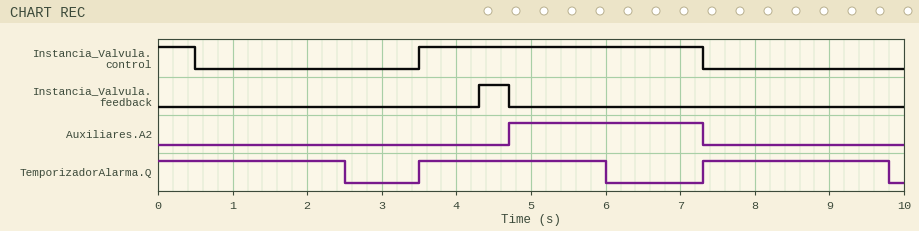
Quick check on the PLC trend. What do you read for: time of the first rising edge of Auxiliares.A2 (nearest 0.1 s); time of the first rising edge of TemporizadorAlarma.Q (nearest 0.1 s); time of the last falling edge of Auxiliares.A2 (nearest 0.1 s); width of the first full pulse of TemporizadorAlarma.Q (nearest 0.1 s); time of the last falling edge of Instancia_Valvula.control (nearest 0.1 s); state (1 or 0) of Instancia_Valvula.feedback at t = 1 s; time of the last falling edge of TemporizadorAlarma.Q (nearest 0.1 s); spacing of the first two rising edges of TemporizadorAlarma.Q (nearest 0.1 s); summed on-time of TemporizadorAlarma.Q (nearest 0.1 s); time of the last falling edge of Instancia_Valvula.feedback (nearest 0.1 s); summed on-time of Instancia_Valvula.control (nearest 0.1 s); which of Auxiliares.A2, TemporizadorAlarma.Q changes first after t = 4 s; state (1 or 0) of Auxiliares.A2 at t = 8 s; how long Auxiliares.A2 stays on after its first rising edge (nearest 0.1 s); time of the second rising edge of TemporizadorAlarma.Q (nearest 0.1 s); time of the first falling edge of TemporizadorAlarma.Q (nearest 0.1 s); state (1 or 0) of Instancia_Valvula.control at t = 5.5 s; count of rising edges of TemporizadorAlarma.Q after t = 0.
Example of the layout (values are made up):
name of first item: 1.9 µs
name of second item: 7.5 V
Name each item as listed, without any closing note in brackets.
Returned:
time of the first rising edge of Auxiliares.A2: 4.7 s
time of the first rising edge of TemporizadorAlarma.Q: 3.5 s
time of the last falling edge of Auxiliares.A2: 7.3 s
width of the first full pulse of TemporizadorAlarma.Q: 2.5 s
time of the last falling edge of Instancia_Valvula.control: 7.3 s
state (1 or 0) of Instancia_Valvula.feedback at t = 1 s: 0
time of the last falling edge of TemporizadorAlarma.Q: 9.8 s
spacing of the first two rising edges of TemporizadorAlarma.Q: 3.8 s
summed on-time of TemporizadorAlarma.Q: 7.5 s
time of the last falling edge of Instancia_Valvula.feedback: 4.7 s
summed on-time of Instancia_Valvula.control: 4.3 s
which of Auxiliares.A2, TemporizadorAlarma.Q changes first after t = 4 s: Auxiliares.A2
state (1 or 0) of Auxiliares.A2 at t = 8 s: 0
how long Auxiliares.A2 stays on after its first rising edge: 2.6 s
time of the second rising edge of TemporizadorAlarma.Q: 7.3 s
time of the first falling edge of TemporizadorAlarma.Q: 2.5 s
state (1 or 0) of Instancia_Valvula.control at t = 5.5 s: 1
count of rising edges of TemporizadorAlarma.Q after t = 0: 2
